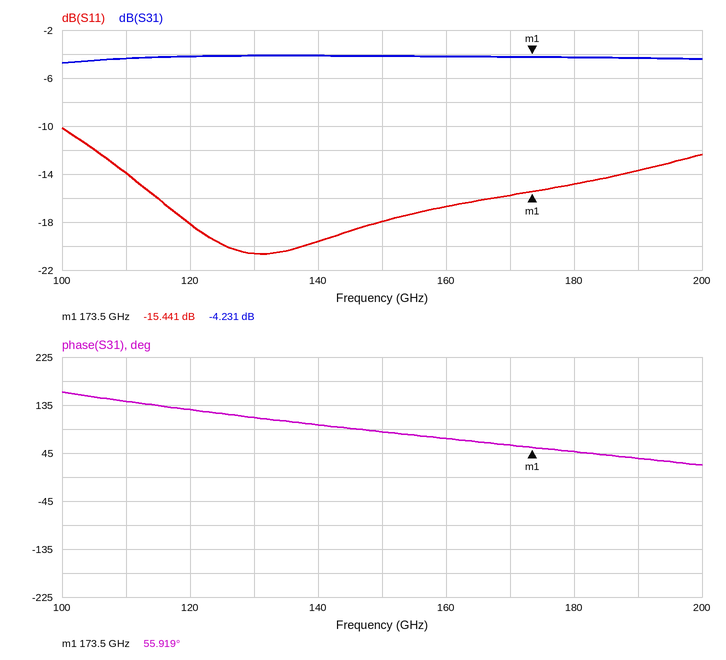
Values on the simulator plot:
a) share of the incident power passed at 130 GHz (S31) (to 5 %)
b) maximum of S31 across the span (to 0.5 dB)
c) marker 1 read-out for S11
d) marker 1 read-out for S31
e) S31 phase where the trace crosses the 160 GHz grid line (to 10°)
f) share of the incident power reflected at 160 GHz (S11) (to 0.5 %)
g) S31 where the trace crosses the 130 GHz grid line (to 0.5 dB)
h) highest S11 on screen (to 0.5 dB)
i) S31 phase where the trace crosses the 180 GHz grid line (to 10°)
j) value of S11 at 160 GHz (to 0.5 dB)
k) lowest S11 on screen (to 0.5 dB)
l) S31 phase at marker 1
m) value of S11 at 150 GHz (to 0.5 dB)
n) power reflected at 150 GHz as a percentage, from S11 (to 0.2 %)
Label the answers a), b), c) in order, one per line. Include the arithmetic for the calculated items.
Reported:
a) 10^(-4/10) ≈ 40 %
b) -4.0 dB
c) -15.441 dB
d) -4.231 dB
e) 70°
f) 10^(-16.5/10) ≈ 2.24 %, so 2.0 % to the nearest 0.5 %
g) -4.0 dB
h) -10.0 dB
i) 50°
j) -16.5 dB
k) -20.5 dB
l) 55.919°
m) -18.0 dB
n) 10^(-18/10) ≈ 1.6 %
